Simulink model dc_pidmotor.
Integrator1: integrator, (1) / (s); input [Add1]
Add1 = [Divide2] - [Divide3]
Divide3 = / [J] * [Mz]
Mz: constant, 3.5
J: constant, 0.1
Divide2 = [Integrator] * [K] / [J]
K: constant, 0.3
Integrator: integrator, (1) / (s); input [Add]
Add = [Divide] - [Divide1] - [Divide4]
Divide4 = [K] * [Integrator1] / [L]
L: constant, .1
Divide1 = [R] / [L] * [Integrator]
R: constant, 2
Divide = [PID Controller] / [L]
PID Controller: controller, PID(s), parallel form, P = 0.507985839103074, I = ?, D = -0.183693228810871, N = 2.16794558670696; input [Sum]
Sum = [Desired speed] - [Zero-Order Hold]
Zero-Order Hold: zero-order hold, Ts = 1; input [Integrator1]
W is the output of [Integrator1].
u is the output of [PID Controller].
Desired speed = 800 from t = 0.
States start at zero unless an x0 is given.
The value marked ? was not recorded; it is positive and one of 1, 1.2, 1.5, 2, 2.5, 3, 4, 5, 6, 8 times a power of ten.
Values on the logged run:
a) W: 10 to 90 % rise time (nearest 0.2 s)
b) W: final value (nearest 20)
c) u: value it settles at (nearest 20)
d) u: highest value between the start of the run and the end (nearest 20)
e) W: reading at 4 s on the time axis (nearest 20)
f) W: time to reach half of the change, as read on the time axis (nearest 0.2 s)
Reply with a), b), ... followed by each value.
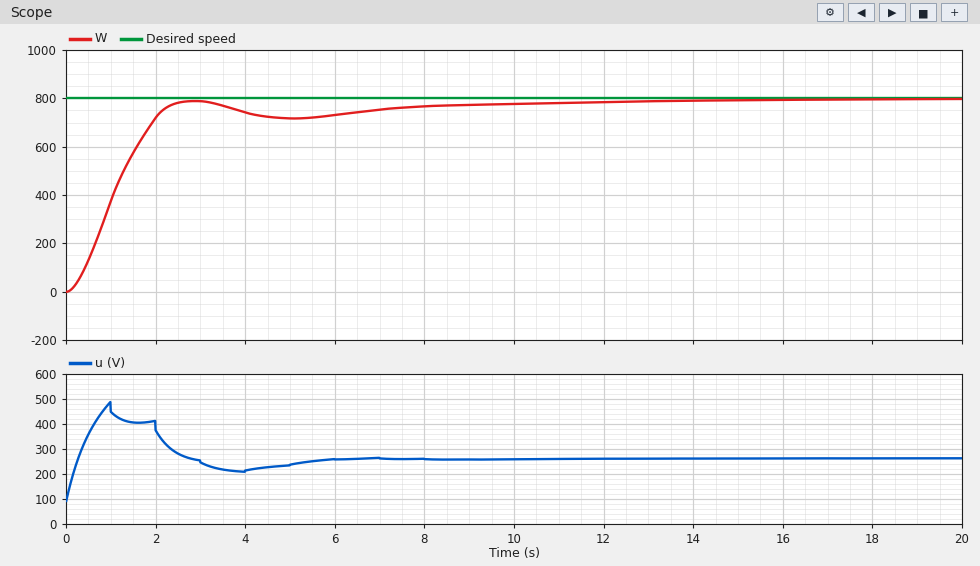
a) 1.6 s
b) 800
c) 260
d) 480
e) 740
f) 1.0 s
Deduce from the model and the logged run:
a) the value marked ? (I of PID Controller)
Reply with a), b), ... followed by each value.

a) 0.15
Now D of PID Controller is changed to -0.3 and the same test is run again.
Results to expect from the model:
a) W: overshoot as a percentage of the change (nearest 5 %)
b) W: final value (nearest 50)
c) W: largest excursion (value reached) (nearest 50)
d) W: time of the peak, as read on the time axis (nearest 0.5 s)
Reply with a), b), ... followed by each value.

a) 10 %
b) 800
c) 900
d) 3.0 s
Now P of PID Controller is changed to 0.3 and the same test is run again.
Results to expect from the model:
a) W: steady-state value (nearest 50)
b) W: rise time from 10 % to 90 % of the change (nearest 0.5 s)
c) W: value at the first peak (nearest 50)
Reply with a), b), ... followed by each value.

a) 800
b) 2.0 s
c) 850
